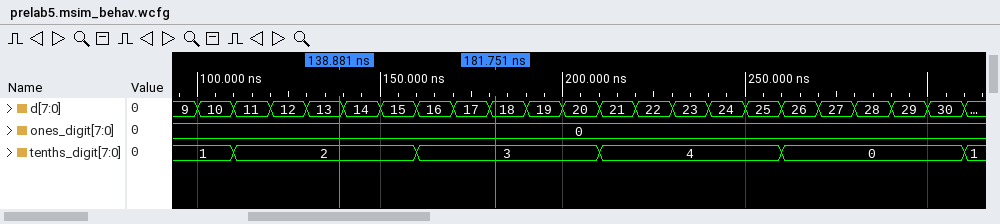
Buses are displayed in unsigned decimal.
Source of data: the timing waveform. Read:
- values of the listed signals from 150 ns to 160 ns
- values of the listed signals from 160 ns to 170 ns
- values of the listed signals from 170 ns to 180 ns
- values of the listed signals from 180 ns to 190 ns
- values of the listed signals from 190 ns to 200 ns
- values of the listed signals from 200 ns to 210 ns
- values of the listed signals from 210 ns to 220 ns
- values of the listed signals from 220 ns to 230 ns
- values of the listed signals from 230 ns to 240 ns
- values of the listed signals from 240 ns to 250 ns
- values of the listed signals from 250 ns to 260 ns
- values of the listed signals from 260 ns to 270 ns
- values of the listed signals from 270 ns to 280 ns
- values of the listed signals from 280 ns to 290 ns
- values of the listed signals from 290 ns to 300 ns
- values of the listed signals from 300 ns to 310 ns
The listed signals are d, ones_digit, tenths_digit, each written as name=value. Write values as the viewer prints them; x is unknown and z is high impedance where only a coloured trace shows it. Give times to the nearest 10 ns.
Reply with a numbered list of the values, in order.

1. d=15, ones_digit=0, tenths_digit=2
2. d=16, ones_digit=0, tenths_digit=3
3. d=17, ones_digit=0, tenths_digit=3
4. d=18, ones_digit=0, tenths_digit=3
5. d=19, ones_digit=0, tenths_digit=3
6. d=20, ones_digit=0, tenths_digit=3
7. d=21, ones_digit=0, tenths_digit=4
8. d=22, ones_digit=0, tenths_digit=4
9. d=23, ones_digit=0, tenths_digit=4
10. d=24, ones_digit=0, tenths_digit=4
11. d=25, ones_digit=0, tenths_digit=4
12. d=26, ones_digit=0, tenths_digit=0
13. d=27, ones_digit=0, tenths_digit=0
14. d=28, ones_digit=0, tenths_digit=0
15. d=29, ones_digit=0, tenths_digit=0
16. d=30, ones_digit=0, tenths_digit=0
